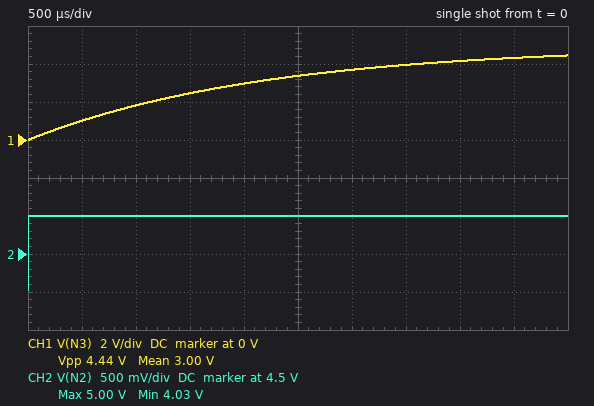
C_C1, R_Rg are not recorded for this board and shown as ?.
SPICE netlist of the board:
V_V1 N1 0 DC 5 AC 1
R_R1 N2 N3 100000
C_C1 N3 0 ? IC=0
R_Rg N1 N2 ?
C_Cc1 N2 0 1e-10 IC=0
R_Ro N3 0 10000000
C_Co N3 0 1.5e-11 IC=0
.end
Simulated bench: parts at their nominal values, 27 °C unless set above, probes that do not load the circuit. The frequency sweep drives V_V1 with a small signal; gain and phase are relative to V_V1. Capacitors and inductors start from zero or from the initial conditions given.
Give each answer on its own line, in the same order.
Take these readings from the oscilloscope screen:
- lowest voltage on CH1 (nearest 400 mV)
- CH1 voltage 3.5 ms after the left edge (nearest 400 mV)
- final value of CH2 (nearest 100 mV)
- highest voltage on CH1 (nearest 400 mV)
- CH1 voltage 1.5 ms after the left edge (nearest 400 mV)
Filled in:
0 V
4.0 V
5.0 V
4.4 V
2.4 V
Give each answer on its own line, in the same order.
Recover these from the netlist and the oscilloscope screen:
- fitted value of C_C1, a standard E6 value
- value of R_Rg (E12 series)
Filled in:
22 nF
120 Ω
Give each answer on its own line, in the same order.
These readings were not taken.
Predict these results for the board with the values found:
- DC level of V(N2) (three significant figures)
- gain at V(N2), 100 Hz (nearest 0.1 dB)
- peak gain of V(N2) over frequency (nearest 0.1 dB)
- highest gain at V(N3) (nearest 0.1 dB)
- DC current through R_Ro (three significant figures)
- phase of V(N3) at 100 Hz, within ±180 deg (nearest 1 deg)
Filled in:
5.00 V
0 dB
0 dB
-0.1 dB
495 nA
-54 deg
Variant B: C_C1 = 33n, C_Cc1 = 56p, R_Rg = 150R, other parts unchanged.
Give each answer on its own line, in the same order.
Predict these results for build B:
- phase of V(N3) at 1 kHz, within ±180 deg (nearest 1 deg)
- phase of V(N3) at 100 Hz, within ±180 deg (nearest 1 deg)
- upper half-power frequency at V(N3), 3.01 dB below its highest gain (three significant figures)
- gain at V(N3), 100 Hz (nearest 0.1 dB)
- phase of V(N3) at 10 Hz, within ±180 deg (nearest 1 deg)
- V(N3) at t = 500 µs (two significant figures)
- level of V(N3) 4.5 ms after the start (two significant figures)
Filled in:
-87 deg
-64 deg
48.6 Hz
-7.3 dB
-12 deg
700 mV
3.7 V
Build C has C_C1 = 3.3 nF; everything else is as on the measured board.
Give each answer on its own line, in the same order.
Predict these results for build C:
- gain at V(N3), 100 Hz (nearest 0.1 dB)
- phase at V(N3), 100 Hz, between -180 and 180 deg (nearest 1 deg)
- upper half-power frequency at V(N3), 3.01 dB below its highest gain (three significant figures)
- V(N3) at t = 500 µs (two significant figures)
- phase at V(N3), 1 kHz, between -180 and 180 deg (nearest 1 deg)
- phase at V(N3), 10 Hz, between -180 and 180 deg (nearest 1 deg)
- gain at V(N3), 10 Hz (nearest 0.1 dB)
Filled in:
-0.3 dB
-12 deg
484 Hz
3.9 V
-64 deg
-1 deg
-0.1 dB
